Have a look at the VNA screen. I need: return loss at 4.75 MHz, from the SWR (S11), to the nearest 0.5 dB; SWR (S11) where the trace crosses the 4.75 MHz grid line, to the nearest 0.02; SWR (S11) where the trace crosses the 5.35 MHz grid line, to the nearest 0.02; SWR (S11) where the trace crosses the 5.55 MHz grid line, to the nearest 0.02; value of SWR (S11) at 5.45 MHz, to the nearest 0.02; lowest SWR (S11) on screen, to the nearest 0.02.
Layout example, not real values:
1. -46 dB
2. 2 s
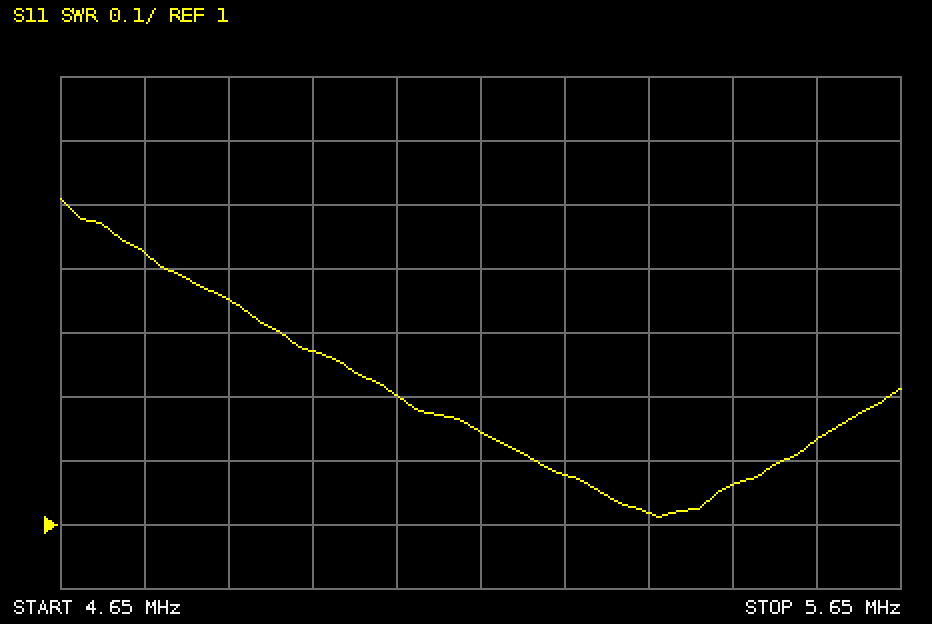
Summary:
1. 15.0 dB
2. 1.42
3. 1.02
4. 1.14
5. 1.06
6. 1.02
